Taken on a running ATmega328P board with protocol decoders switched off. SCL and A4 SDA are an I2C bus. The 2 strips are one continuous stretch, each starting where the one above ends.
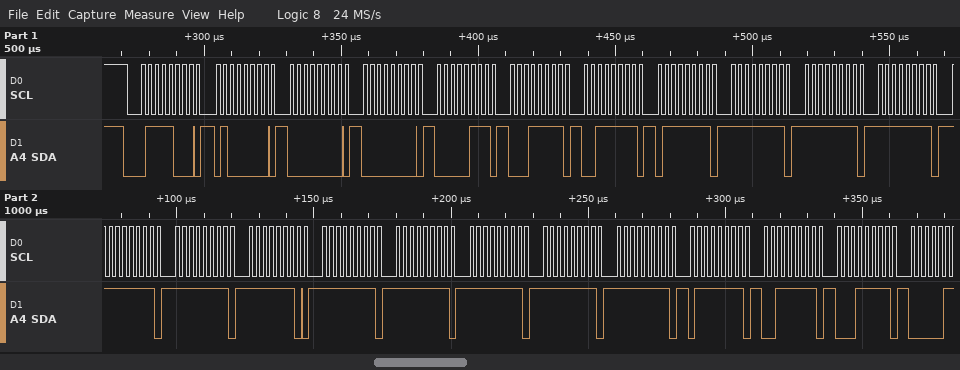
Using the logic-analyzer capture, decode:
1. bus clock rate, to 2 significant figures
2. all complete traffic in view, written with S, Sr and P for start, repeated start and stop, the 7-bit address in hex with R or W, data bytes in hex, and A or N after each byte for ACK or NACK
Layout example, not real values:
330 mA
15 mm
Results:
400 kHz
S 3CW A 40 A 00 A 00 A 07 A 1F A 3F A 7F A FF A FF A FF A FF A FF A FE A FF A FF A FF A FF A FF A 7F A 3F A 1F A
